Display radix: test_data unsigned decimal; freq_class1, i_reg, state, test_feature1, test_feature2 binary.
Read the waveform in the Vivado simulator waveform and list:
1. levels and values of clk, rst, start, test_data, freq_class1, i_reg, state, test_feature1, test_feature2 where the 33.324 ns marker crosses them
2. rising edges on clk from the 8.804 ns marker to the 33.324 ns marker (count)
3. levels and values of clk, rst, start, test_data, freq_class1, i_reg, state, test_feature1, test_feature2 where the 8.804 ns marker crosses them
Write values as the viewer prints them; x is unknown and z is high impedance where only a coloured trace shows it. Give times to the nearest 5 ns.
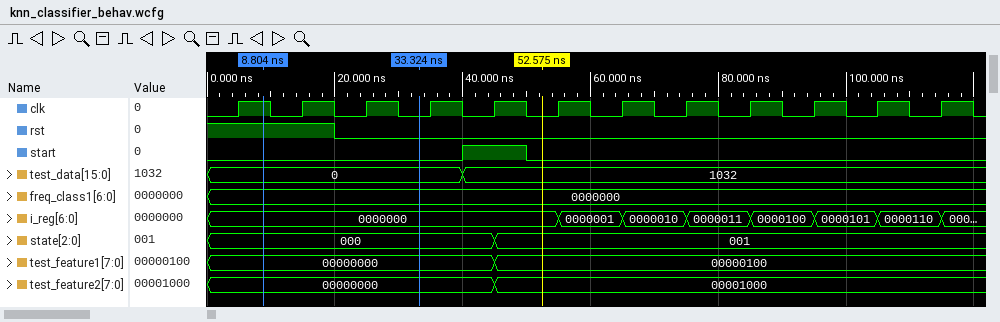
clk=0, rst=0, start=0, test_data=0, freq_class1=0000000, i_reg=0000000, state=000, test_feature1=00000000, test_feature2=00000000
2
clk=1, rst=1, start=0, test_data=0, freq_class1=0000000, i_reg=0000000, state=000, test_feature1=00000000, test_feature2=00000000
